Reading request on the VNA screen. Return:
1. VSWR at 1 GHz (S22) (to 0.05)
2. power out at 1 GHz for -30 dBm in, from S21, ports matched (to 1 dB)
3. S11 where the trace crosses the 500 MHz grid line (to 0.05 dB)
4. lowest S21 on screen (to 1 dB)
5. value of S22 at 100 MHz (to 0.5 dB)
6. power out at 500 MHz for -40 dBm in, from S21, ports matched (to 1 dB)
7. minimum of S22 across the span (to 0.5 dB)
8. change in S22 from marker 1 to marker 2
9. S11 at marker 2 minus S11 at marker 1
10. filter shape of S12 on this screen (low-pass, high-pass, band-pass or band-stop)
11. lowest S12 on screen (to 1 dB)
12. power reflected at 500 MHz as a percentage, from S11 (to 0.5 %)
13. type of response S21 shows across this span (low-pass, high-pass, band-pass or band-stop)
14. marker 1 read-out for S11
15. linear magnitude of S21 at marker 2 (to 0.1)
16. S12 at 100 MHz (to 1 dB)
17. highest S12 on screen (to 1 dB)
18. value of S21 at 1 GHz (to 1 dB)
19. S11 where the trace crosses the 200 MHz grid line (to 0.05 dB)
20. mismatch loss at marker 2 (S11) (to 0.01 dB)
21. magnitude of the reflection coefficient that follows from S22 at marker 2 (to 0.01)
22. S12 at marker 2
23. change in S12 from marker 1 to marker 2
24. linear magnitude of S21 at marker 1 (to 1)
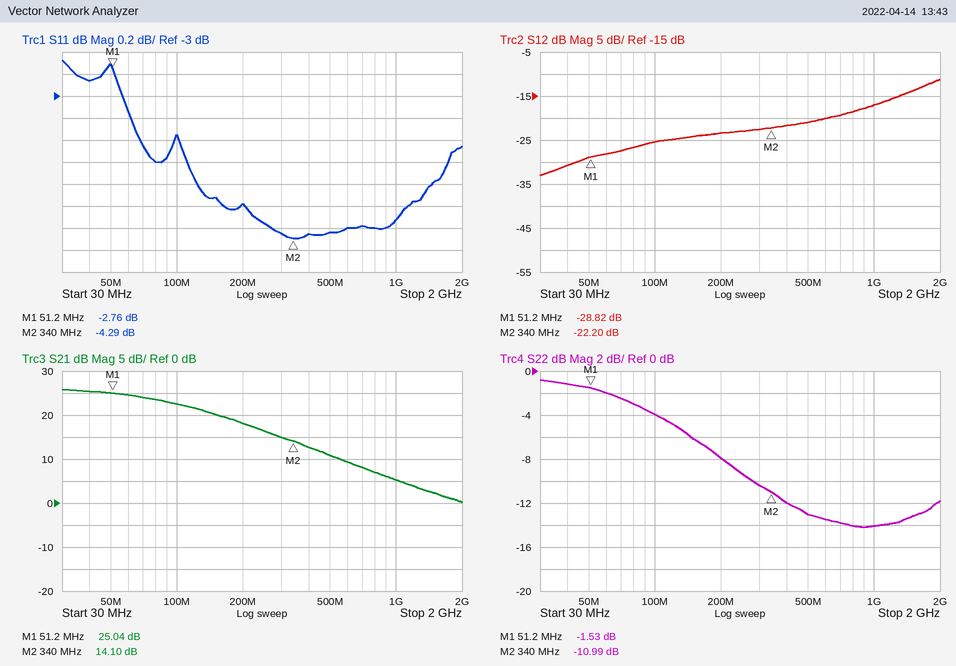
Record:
1.50
-25 dBm
-4.25 dB
0 dB
-4.0 dB
-29 dBm
-14.0 dB
-9.46 dB
-1.53 dB
high-pass
-33 dB
37.5 %
low-pass
-2.76 dB
5.1
-25 dB
-11 dB
5 dB
-4.00 dB
2.02 dB
0.28
-22.20 dB
6.62 dB
18
